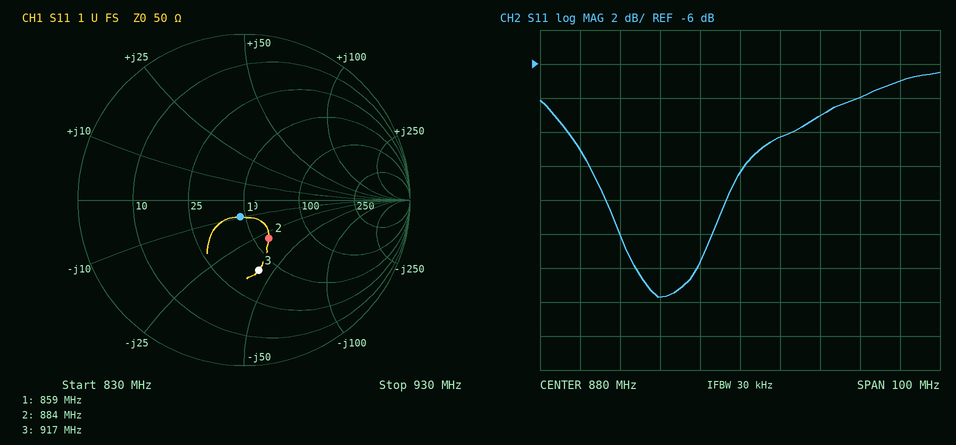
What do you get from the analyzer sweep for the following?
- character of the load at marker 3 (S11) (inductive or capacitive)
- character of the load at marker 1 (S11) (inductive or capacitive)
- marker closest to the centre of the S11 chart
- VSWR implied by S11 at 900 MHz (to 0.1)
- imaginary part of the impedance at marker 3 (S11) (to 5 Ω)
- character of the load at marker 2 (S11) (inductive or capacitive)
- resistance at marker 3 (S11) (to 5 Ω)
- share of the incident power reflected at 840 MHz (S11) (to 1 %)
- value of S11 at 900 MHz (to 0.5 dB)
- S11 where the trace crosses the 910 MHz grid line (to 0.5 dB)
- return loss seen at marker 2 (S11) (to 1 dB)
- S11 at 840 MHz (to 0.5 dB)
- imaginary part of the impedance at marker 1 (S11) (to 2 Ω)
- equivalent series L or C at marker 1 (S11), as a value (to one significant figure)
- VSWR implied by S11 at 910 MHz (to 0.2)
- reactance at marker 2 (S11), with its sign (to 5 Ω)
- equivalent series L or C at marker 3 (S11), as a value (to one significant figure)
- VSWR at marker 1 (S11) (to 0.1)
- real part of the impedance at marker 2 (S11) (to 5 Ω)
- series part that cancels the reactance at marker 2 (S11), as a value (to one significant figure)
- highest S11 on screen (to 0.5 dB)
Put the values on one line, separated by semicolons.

capacitive; capacitive; marker 1; 2.1; -40 Ω; capacitive; 40 Ω; 8 %; -9.0 dB; -8.0 dB; 11 dB; -11.0 dB; -10 Ω; 20 pF; 2.4; -30 Ω; 4 pF; 1.2; 60 Ω; 5 nH; -6.5 dB
